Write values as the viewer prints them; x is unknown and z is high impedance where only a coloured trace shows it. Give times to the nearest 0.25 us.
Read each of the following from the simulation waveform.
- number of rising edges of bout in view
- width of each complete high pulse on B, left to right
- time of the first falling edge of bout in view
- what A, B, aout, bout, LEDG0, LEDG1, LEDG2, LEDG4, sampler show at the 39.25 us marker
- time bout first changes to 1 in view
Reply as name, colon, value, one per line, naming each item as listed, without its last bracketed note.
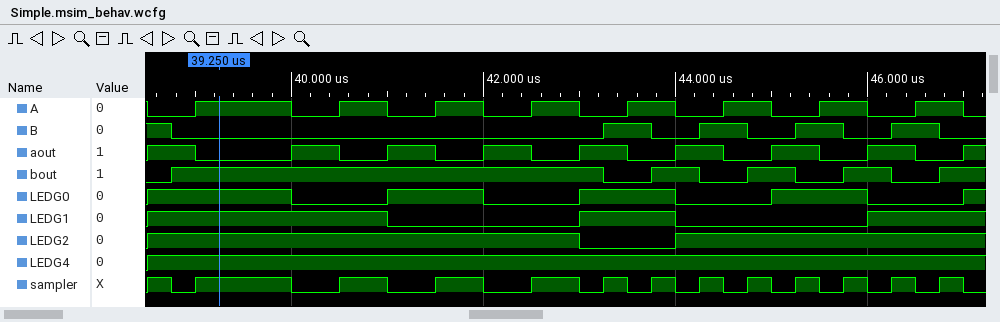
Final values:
number of rising edges of bout in view: 5
width of each complete high pulse on B, left to right: 0.5 us, 0.5 us, 0.5 us, 0.5 us
time of the first falling edge of bout in view: 43.25 us
what A, B, aout, bout, LEDG0, LEDG1, LEDG2, LEDG4, sampler show at the 39.25 us marker: A=1, B=0, aout=0, bout=1, LEDG0=1, LEDG1=1, LEDG2=1, LEDG4=1, sampler=1
time bout first changes to 1 in view: 38.75 us
